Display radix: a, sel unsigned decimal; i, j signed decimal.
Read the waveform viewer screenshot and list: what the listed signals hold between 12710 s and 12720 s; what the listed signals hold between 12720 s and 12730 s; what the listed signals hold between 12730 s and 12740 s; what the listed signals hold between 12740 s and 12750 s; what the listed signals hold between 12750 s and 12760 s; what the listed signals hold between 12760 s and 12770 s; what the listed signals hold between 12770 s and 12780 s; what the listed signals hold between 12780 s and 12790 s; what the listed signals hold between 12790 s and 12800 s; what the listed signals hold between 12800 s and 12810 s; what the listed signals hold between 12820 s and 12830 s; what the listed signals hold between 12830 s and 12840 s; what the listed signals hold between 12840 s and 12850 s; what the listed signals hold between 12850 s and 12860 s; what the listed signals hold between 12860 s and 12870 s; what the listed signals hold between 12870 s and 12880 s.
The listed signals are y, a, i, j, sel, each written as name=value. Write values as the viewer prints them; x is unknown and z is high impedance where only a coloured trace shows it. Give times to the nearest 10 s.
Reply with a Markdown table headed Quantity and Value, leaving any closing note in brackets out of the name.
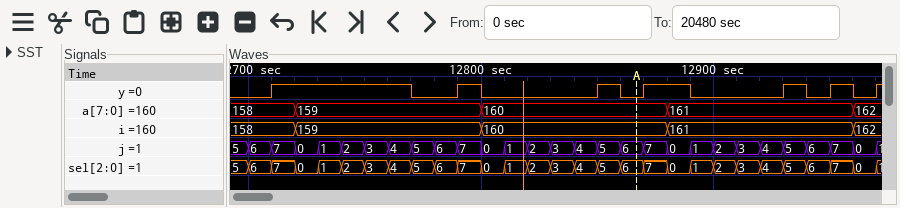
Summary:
| Quantity | Value |
|---|---|
| what the listed signals hold between 12710 s and 12720 s | y=1, a=158, i=158, j=7, sel=7 |
| what the listed signals hold between 12720 s and 12730 s | y=1, a=159, i=159, j=0, sel=0 |
| what the listed signals hold between 12730 s and 12740 s | y=1, a=159, i=159, j=1, sel=1 |
| what the listed signals hold between 12740 s and 12750 s | y=1, a=159, i=159, j=2, sel=2 |
| what the listed signals hold between 12750 s and 12760 s | y=1, a=159, i=159, j=3, sel=3 |
| what the listed signals hold between 12760 s and 12770 s | y=1, a=159, i=159, j=4, sel=4 |
| what the listed signals hold between 12770 s and 12780 s | y=0, a=159, i=159, j=5, sel=5 |
| what the listed signals hold between 12780 s and 12790 s | y=0, a=159, i=159, j=6, sel=6 |
| what the listed signals hold between 12790 s and 12800 s | y=1, a=159, i=159, j=7, sel=7 |
| what the listed signals hold between 12800 s and 12810 s | y=0, a=160, i=160, j=0, sel=0 |
| what the listed signals hold between 12820 s and 12830 s | y=0, a=160, i=160, j=2, sel=2 |
| what the listed signals hold between 12830 s and 12840 s | y=0, a=160, i=160, j=3, sel=3 |
| what the listed signals hold between 12840 s and 12850 s | y=0, a=160, i=160, j=4, sel=4 |
| what the listed signals hold between 12850 s and 12860 s | y=1, a=160, i=160, j=5, sel=5 |
| what the listed signals hold between 12860 s and 12870 s | y=0, a=160, i=160, j=6, sel=6 |
| what the listed signals hold between 12870 s and 12880 s | y=1, a=160, i=160, j=7, sel=7 |
